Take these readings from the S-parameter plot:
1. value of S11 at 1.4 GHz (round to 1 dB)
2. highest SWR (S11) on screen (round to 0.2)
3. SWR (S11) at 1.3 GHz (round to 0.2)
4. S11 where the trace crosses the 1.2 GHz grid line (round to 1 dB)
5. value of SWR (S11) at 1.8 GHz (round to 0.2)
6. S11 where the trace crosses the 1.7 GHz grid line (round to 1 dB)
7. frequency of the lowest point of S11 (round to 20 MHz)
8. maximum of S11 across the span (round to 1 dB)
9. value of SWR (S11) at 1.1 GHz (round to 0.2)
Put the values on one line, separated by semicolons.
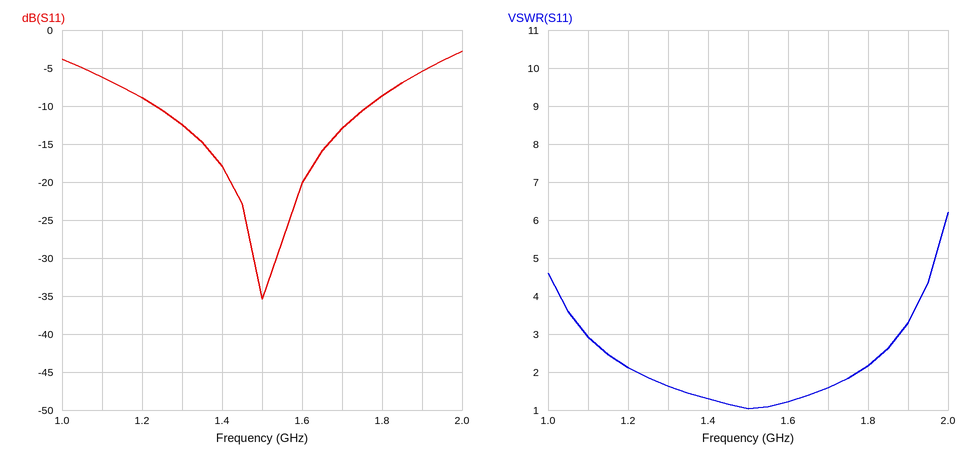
-18 dB; 6.2; 1.6; -9 dB; 2.2; -13 dB; 1.50 GHz; -3 dB; 3.0
